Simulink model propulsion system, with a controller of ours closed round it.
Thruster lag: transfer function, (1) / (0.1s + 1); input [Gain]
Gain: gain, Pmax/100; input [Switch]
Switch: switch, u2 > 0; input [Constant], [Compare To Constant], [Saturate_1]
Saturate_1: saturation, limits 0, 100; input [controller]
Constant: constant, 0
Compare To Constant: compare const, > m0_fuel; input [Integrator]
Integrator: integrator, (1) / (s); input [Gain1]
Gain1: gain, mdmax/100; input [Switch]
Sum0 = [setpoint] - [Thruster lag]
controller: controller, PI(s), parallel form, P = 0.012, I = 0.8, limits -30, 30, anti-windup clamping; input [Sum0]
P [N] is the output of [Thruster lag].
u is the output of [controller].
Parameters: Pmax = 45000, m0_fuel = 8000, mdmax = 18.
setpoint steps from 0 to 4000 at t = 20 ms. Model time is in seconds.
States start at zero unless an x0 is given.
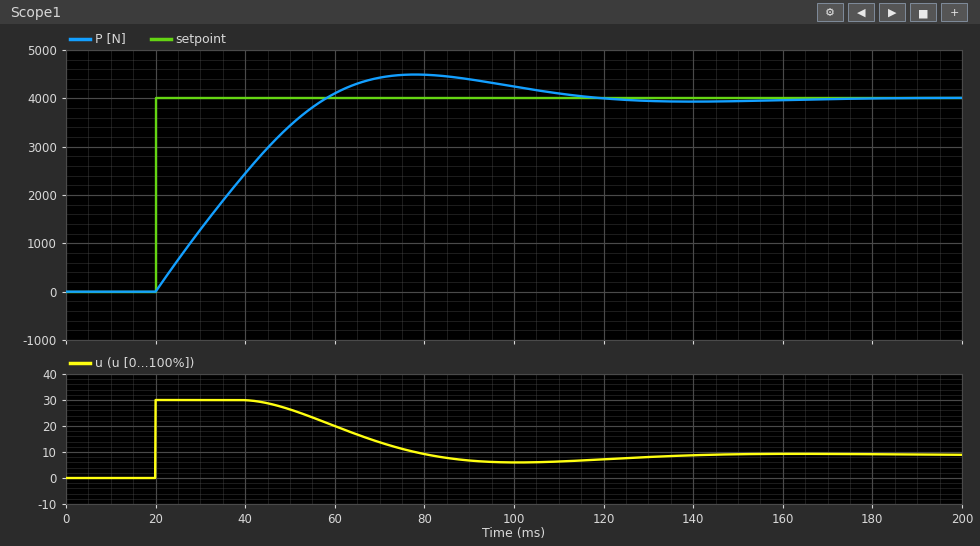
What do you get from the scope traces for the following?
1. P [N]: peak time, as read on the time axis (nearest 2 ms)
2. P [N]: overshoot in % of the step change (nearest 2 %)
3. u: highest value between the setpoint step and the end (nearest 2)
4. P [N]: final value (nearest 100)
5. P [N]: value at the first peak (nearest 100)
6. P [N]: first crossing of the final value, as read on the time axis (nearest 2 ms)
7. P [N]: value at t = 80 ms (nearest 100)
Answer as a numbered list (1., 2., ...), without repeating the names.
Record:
1. 78 ms
2. 12 %
3. 30
4. 4000
5. 4500
6. 58 ms
7. 4500
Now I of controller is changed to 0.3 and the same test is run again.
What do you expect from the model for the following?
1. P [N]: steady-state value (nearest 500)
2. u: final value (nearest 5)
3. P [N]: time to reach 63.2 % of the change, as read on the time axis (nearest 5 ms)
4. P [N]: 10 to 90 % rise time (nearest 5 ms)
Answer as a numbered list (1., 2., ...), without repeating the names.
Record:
1. 4000
2. 10
3. 40 ms
4. 40 ms
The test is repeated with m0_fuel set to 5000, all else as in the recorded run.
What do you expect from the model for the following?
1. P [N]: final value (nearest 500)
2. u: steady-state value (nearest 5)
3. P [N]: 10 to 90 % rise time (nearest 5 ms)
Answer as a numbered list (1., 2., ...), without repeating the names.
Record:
1. 4000
2. 10
3. 30 ms
